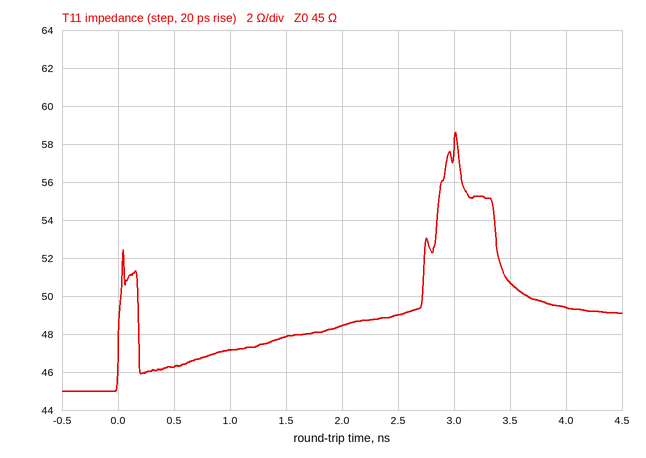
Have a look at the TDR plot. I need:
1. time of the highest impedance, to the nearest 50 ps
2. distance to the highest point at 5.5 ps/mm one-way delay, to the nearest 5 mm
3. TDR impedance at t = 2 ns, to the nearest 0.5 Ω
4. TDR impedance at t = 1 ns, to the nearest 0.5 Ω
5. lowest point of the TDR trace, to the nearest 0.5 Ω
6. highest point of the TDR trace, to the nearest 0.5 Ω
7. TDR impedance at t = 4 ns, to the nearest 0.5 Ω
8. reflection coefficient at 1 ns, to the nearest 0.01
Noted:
3.00 ns
275 mm
48.5 Ω
47.0 Ω
45.0 Ω
58.5 Ω
49.5 Ω
+0.02
